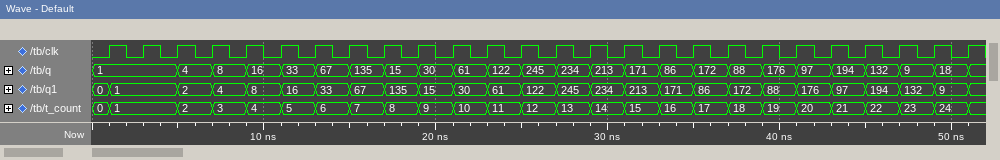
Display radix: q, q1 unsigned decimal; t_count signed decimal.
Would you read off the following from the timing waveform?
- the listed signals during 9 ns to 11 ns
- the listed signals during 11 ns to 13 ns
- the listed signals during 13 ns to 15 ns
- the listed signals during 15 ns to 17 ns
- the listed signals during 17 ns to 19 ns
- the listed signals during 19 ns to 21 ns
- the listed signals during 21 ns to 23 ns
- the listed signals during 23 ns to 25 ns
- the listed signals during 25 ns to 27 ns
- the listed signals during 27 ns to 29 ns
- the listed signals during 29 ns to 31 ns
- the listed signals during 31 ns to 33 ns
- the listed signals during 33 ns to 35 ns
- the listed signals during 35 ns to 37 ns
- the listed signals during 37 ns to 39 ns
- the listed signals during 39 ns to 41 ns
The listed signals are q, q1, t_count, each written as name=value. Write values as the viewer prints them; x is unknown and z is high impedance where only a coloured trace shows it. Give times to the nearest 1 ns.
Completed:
q=16, q1=8, t_count=4
q=33, q1=16, t_count=5
q=67, q1=33, t_count=6
q=135, q1=67, t_count=7
q=15, q1=135, t_count=8
q=30, q1=15, t_count=9
q=61, q1=30, t_count=10
q=122, q1=61, t_count=11
q=245, q1=122, t_count=12
q=234, q1=245, t_count=13
q=213, q1=234, t_count=14
q=171, q1=213, t_count=15
q=86, q1=171, t_count=16
q=172, q1=86, t_count=17
q=88, q1=172, t_count=18
q=176, q1=88, t_count=19
